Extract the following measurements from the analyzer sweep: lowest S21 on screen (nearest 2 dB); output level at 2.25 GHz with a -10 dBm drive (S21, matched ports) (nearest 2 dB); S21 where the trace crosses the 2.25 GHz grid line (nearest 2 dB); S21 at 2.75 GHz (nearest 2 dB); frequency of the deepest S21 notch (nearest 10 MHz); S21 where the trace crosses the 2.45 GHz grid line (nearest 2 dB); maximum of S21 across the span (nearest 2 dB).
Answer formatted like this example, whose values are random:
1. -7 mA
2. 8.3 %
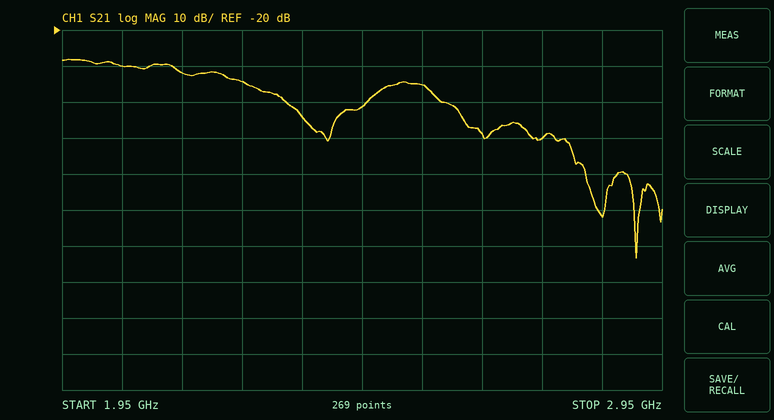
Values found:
1. -84 dB
2. -44 dBm
3. -34 dB
4. -50 dB
5. 2.91 GHz
6. -42 dB
7. -28 dB
